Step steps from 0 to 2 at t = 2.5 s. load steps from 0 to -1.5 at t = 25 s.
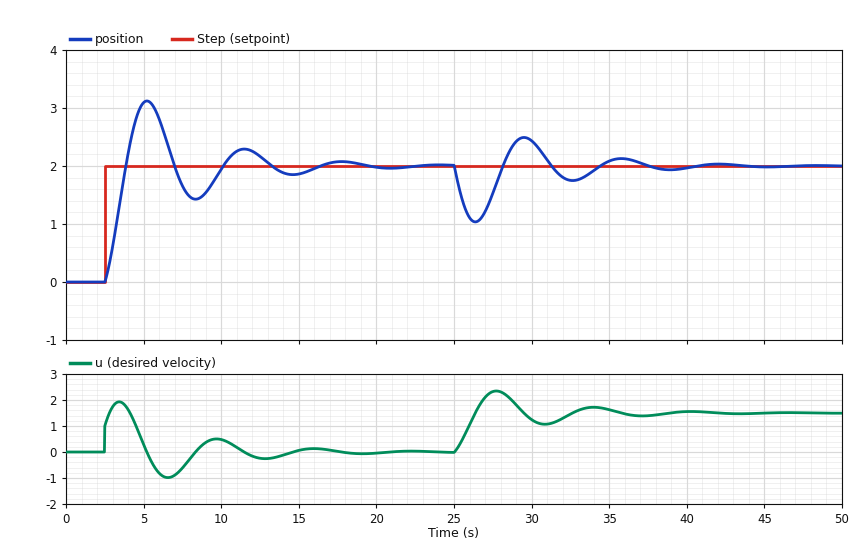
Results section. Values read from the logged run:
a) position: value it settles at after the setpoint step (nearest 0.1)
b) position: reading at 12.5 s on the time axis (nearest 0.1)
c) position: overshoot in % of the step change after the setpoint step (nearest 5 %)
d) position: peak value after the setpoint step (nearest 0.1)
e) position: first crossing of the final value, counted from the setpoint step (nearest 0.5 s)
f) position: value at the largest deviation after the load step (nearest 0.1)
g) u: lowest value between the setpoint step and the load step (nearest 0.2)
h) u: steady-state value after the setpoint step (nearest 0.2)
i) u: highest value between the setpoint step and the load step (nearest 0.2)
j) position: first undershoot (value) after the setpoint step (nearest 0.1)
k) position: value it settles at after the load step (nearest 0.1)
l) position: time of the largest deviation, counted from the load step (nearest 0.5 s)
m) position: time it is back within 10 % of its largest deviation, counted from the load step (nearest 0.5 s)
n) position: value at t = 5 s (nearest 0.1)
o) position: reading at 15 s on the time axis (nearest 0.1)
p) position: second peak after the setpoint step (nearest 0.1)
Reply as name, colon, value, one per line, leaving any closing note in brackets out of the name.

position: value it settles at after the setpoint step: 2.0
position: reading at 12.5 s on the time axis: 2.2
position: overshoot in % of the step change after the setpoint step: 55 %
position: peak value after the setpoint step: 3.1
position: first crossing of the final value, counted from the setpoint step: 1.5 s
position: value at the largest deviation after the load step: 1.0
u: lowest value between the setpoint step and the load step: -1.0
u: steady-state value after the setpoint step: 0.0
u: highest value between the setpoint step and the load step: 2.0
position: first undershoot (value) after the setpoint step: 1.4
position: value it settles at after the load step: 2.0
position: time of the largest deviation, counted from the load step: 1.5 s
position: time it is back within 10 % of its largest deviation, counted from the load step: 11.5 s
position: value at t = 5 s: 3.1
position: reading at 15 s on the time axis: 1.9
position: second peak after the setpoint step: 2.3
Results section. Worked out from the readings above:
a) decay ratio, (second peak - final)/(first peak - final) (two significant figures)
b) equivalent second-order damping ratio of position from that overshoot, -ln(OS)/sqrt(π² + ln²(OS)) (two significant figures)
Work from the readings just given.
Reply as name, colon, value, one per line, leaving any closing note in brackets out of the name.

decay ratio, (second peak - final)/(first peak - final): 0.27
equivalent second-order damping ratio of position from that overshoot, -ln(OS)/sqrt(π² + ln²(OS)): 0.19
